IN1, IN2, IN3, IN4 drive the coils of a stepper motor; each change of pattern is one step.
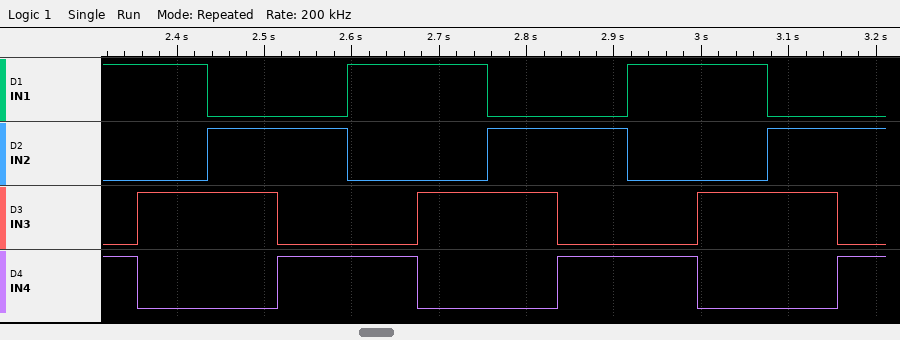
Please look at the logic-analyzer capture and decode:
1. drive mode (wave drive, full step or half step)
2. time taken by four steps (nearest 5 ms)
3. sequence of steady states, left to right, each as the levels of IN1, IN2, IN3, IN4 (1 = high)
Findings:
full step
320 ms
1001 1010 0110 0101 1001 1010 0110 0101 1001 1010 0110 0101
